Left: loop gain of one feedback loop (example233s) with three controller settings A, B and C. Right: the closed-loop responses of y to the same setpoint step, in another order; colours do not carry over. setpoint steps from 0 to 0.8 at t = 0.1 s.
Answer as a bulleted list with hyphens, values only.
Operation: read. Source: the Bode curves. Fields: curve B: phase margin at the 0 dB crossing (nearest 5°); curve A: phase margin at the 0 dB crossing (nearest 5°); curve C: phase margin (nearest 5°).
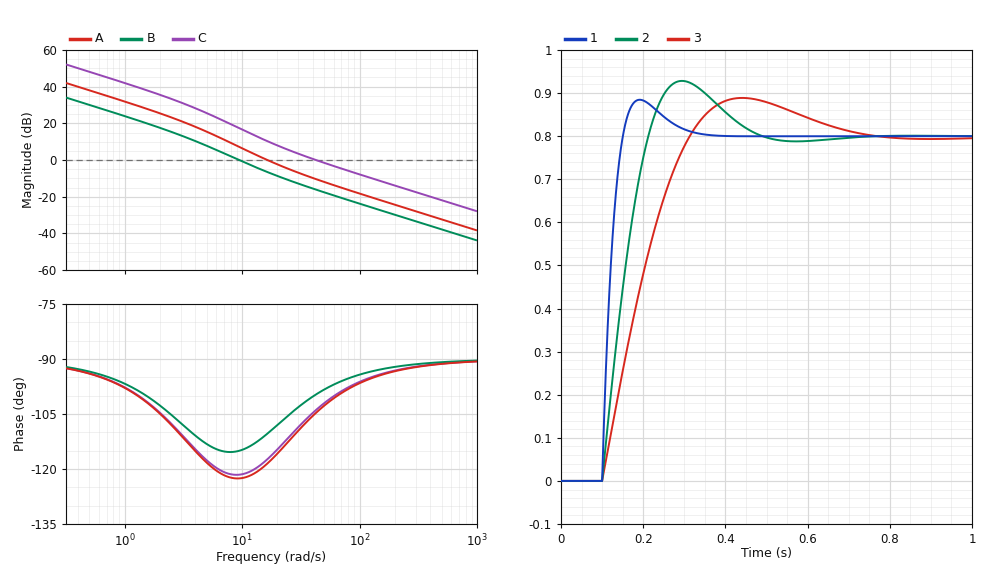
- 65°
- 60°
- 75°
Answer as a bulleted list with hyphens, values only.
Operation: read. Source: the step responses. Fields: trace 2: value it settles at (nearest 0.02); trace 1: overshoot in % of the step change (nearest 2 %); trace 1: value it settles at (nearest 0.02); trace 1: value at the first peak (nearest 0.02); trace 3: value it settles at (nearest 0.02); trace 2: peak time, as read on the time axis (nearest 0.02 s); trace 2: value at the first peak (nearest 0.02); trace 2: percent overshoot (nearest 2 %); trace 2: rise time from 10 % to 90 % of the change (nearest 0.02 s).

- 0.80
- 10 %
- 0.80
- 0.88
- 0.80
- 0.30 s
- 0.92
- 16 %
- 0.08 s
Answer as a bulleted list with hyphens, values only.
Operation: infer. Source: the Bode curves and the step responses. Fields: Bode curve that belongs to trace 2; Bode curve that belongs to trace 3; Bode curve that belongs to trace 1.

- A
- B
- C
